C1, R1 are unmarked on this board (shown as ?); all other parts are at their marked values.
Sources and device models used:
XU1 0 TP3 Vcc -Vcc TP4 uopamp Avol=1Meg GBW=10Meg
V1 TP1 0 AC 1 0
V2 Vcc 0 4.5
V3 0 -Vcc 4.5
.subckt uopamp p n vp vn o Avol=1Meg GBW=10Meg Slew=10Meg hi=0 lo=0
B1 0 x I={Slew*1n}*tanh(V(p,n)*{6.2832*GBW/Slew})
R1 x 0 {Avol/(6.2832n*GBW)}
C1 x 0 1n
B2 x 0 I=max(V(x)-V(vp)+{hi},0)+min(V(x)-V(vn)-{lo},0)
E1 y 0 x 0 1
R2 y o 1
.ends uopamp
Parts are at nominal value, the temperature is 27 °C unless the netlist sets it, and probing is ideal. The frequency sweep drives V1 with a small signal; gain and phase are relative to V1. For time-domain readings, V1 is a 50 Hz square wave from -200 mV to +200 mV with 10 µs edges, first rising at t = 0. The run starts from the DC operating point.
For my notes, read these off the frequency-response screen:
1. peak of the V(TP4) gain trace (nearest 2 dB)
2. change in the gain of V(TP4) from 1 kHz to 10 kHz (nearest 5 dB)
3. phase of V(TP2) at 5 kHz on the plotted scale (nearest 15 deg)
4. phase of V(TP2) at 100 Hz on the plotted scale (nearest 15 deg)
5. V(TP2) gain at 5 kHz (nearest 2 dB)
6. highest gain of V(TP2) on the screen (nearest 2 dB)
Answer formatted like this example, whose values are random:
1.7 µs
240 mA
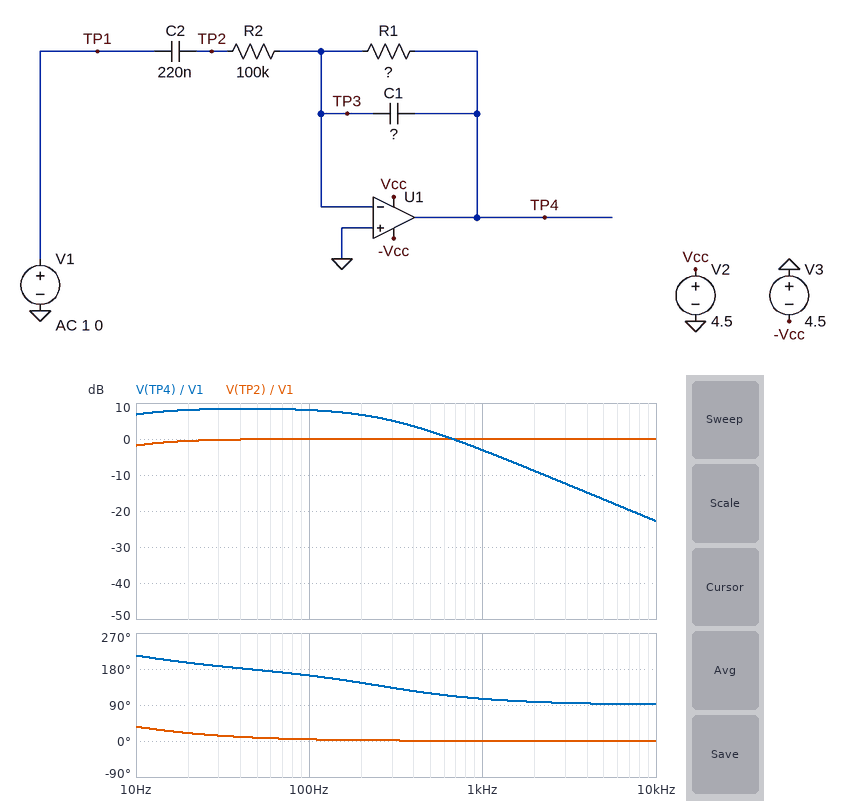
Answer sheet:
8 dB
-20 dB
0 deg
0 deg
0 dB
0 dB
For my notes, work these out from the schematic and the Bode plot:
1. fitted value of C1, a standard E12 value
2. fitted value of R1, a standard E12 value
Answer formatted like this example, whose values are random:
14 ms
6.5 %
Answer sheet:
2.2 nF
270 kΩ
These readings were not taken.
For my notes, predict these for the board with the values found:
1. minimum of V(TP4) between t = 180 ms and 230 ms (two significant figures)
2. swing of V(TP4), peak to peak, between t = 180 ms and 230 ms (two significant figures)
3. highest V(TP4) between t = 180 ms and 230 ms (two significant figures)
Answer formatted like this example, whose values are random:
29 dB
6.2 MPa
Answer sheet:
-590 mV
1.2 V
590 mV
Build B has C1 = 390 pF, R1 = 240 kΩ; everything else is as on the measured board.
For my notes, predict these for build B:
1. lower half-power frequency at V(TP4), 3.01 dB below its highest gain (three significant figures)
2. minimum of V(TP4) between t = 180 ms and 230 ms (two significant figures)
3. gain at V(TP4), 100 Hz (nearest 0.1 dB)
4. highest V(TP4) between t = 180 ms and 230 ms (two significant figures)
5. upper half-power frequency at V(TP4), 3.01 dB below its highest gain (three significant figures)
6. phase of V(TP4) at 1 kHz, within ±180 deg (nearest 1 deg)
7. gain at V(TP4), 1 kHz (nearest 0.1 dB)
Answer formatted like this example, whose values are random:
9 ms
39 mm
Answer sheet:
7.17 Hz
-570 mV
7.6 dB
570 mV
1.71 kHz
150 deg
6.3 dB
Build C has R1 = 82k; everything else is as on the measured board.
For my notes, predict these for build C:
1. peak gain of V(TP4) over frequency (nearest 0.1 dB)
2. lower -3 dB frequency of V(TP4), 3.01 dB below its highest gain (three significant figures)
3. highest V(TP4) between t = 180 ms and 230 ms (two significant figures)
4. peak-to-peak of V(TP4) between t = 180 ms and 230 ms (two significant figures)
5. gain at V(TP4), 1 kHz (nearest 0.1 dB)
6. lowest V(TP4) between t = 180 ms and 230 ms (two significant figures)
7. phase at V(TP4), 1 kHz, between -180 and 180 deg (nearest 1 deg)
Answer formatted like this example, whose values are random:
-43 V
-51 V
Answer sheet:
-1.8 dB
7.12 Hz
190 mV
380 mV
-5.3 dB
-190 mV
132 deg
